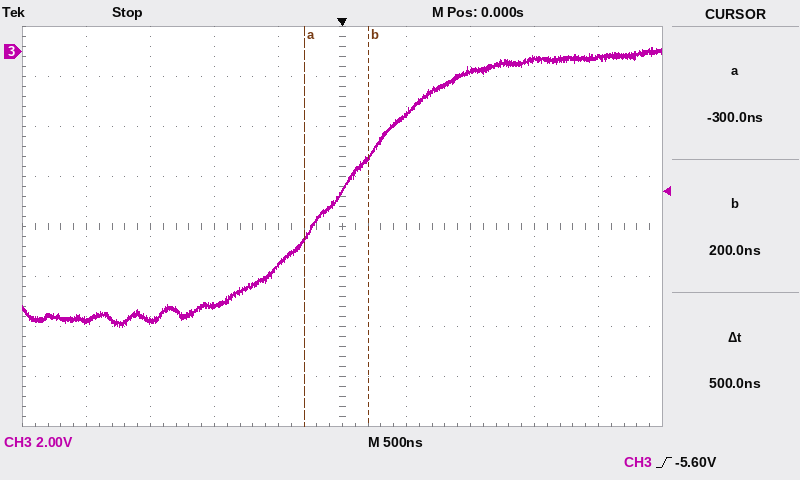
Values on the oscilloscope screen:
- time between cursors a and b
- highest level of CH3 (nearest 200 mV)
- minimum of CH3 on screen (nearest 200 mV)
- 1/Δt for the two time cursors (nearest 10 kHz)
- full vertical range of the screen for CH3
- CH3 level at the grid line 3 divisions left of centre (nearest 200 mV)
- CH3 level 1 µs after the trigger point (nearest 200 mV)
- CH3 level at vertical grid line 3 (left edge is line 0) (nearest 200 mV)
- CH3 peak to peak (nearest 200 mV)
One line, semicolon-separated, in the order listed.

500 ns; 200 mV; -11.0 V; 2.00 MHz; 16 V; -10.8 V; -800 mV; -10.2 V; 11.2 V
